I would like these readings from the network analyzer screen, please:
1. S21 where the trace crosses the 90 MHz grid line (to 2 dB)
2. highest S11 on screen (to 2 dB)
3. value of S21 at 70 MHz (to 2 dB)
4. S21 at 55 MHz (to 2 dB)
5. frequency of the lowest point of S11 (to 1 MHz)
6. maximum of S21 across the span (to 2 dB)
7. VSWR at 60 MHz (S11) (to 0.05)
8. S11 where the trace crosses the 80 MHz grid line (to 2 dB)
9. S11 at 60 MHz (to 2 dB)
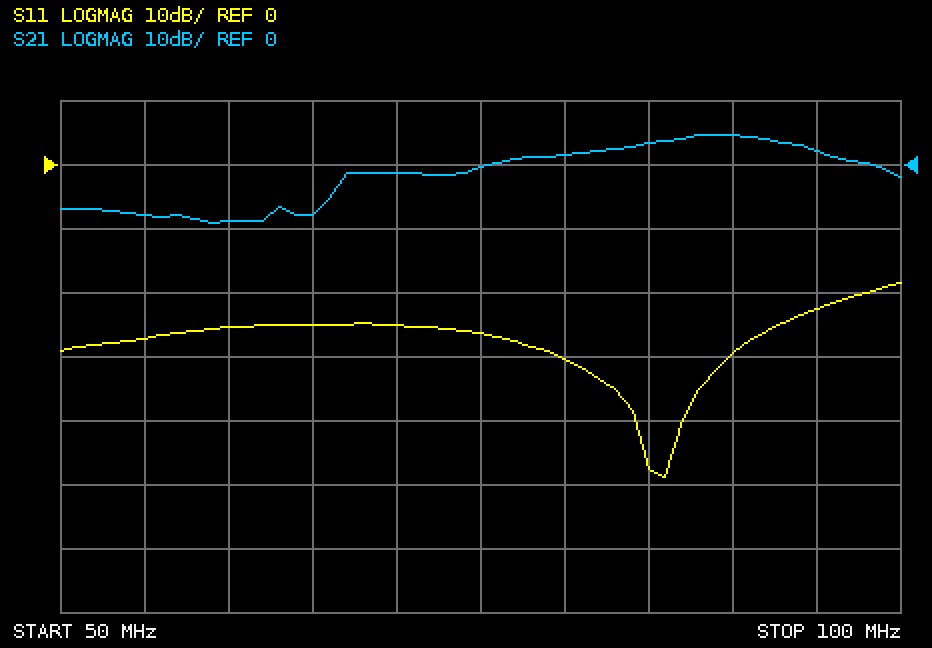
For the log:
4 dB
-18 dB
-2 dB
-8 dB
86 MHz
4 dB
1.10
-30 dB
-26 dB
